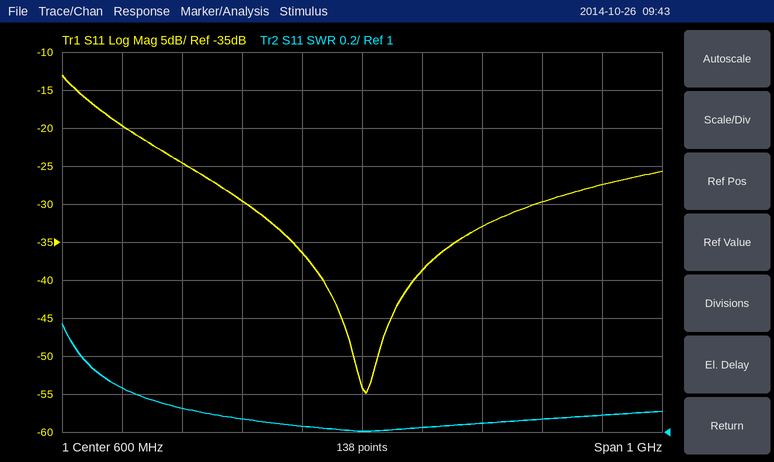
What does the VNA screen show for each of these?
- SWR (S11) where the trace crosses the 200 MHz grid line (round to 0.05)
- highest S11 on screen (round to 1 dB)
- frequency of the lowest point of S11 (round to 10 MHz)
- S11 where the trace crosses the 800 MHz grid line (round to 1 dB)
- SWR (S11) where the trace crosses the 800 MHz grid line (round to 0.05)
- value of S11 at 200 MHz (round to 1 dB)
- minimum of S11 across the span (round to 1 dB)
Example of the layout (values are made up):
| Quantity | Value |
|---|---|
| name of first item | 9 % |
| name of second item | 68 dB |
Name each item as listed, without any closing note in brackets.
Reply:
| Quantity | Value |
|---|---|
| SWR (S11) where the trace crosses the 200 MHz grid line | 1.25 |
| highest S11 on screen | -13 dB |
| frequency of the lowest point of S11 | 610 MHz |
| S11 where the trace crosses the 800 MHz grid line | -33 dB |
| SWR (S11) where the trace crosses the 800 MHz grid line | 1.05 |
| value of S11 at 200 MHz | -20 dB |
| minimum of S11 across the span | -55 dB |
